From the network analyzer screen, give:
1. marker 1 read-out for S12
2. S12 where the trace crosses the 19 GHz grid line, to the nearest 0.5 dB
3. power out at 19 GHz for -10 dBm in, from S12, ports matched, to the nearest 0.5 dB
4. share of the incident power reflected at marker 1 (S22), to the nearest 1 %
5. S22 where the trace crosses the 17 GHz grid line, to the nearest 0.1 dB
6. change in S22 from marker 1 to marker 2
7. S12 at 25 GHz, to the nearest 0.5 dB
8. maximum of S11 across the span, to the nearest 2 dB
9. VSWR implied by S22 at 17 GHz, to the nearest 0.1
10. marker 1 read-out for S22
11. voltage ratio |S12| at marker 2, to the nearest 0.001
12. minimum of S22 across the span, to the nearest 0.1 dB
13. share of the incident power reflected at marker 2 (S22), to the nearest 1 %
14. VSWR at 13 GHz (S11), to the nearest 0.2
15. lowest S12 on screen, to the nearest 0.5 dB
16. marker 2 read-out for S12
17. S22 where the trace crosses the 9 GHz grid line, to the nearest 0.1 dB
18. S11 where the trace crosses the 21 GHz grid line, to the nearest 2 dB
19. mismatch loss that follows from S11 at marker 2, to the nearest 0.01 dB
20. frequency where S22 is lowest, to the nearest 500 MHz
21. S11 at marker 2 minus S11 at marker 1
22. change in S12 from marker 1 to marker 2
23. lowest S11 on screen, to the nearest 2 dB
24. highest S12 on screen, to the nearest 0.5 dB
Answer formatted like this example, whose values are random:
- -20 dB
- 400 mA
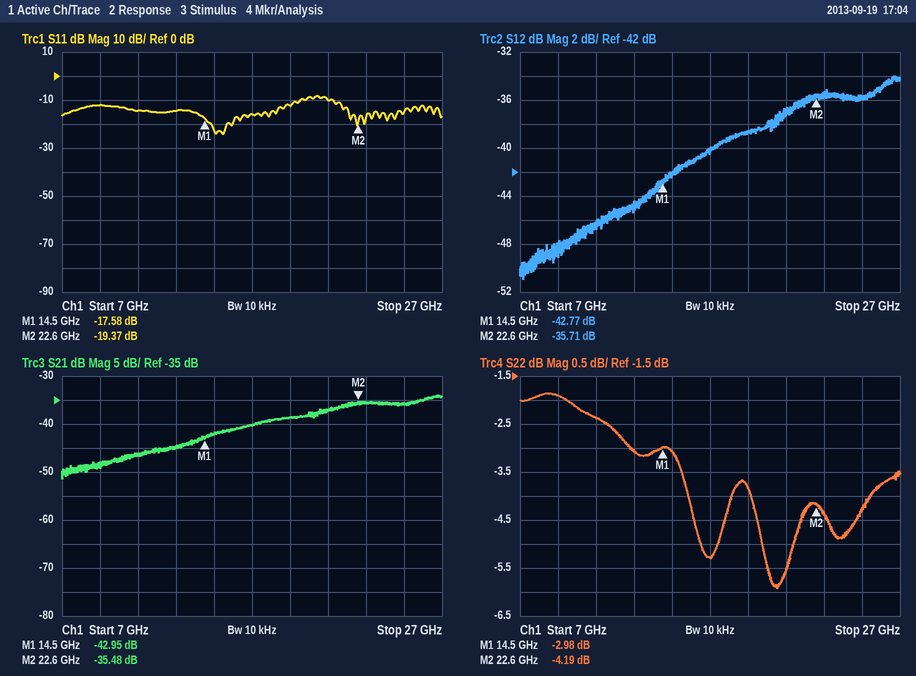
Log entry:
- -42.77 dB
- -38.5 dB
- -48.5 dBm
- 50 %
- -5.3 dB
- -1.21 dB
- -36.0 dB
- -8 dB
- 3.4
- -2.98 dB
- 0.016
- -5.9 dB
- 38 %
- 1.4
- -51.0 dB
- -35.71 dB
- -1.9 dB
- -10 dB
- 0.05 dB
- 20.5 GHz
- -1.79 dB
- 7.06 dB
- -24 dB
- -34.0 dB
